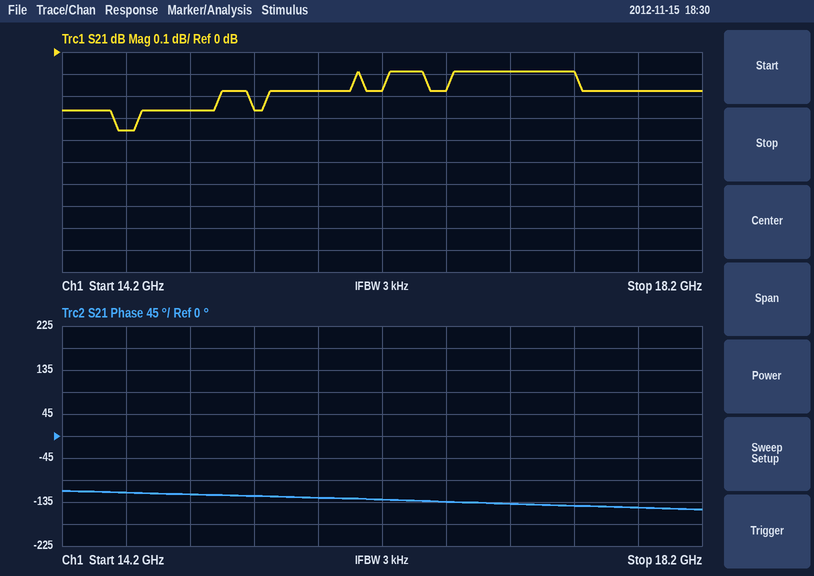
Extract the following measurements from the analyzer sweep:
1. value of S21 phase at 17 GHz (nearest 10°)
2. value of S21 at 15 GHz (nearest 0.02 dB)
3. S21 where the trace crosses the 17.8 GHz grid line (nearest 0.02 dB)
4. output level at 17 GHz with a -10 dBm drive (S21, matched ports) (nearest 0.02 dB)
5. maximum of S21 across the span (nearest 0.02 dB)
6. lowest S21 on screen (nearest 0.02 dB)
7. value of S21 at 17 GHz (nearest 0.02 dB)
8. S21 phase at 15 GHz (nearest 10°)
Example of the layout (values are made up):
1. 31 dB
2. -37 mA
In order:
1. -140°
2. -0.26 dB
3. -0.18 dB
4. -10.08 dBm
5. -0.08 dB
6. -0.36 dB
7. -0.08 dB
8. -120°
